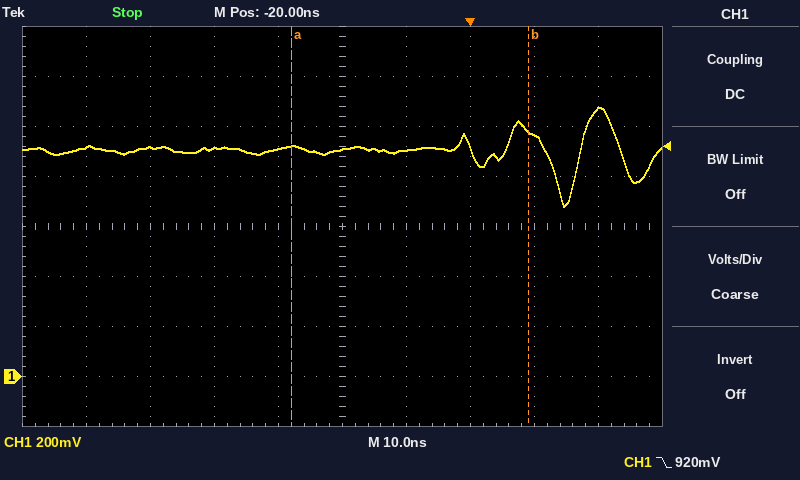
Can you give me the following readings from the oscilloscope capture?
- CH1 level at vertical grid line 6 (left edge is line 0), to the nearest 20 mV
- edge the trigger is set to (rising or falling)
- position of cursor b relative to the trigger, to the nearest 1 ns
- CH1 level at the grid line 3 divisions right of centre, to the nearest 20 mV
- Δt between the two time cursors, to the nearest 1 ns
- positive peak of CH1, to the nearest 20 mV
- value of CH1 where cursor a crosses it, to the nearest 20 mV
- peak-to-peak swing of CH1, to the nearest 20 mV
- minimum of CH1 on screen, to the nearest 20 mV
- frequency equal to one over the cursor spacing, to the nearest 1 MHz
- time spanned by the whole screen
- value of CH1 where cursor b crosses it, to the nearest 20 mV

900 mV
falling
+9 ns
960 mV
37 ns
1.08 V
920 mV
400 mV
680 mV
27 MHz
100 ns
980 mV
